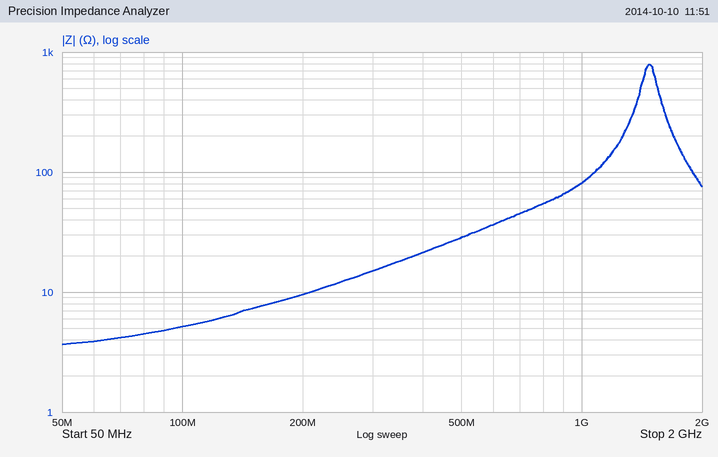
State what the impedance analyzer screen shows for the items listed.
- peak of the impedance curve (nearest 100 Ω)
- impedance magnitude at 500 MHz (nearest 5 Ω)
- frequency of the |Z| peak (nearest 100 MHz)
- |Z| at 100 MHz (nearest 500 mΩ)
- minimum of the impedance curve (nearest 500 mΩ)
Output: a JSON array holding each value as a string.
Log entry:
["800 Ω", "30 Ω", "1.5 GHz", "5.0 Ω", "3.5 Ω"]
